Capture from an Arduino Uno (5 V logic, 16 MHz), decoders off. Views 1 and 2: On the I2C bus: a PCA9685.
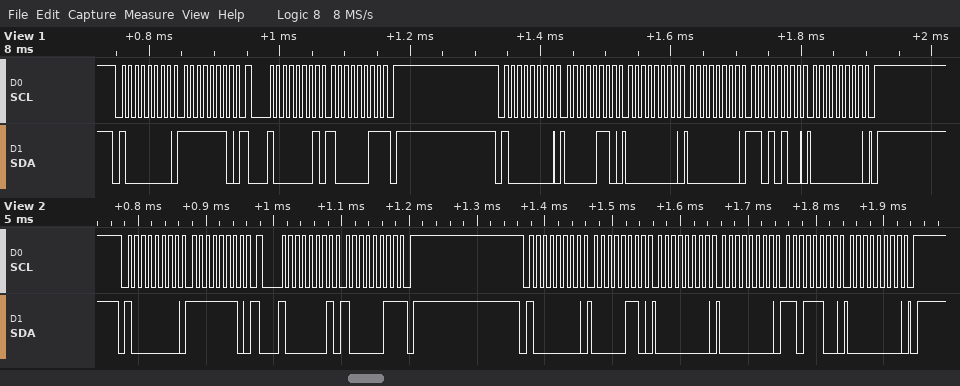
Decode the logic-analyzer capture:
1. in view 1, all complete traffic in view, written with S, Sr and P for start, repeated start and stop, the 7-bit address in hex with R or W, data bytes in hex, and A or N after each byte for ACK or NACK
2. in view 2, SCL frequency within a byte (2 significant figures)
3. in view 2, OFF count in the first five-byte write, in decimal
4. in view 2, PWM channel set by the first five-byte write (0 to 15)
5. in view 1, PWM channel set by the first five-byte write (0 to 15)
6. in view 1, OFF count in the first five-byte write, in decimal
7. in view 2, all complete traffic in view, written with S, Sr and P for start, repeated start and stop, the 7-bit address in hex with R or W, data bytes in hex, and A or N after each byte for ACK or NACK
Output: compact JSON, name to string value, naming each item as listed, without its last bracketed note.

{"in view 1, all complete traffic in view, written with S, Sr and P for start, repeated start and stop, the 7-bit address in hex with R or W, data bytes in hex, and A or N after each byte for ACK or NACK": "S 40W A FE A Sr 40R A 83 N P S 40W A 06 A 00 A 00 A D4 A 00 A P", "in view 2, SCL frequency within a byte": "100 kHz", "in view 2, OFF count in the first five-byte write, in decimal": "220", "in view 2, PWM channel set by the first five-byte write": "0", "in view 1, PWM channel set by the first five-byte write": "0", "in view 1, OFF count in the first five-byte write, in decimal": "212", "in view 2, all complete traffic in view, written with S, Sr and P for start, repeated start and stop, the 7-bit address in hex with R or W, data bytes in hex, and A or N after each byte for ACK or NACK": "S 40W A FE A Sr 40R A 83 N P S 40W A 06 A 00 A 00 A DC A 00 A P"}
